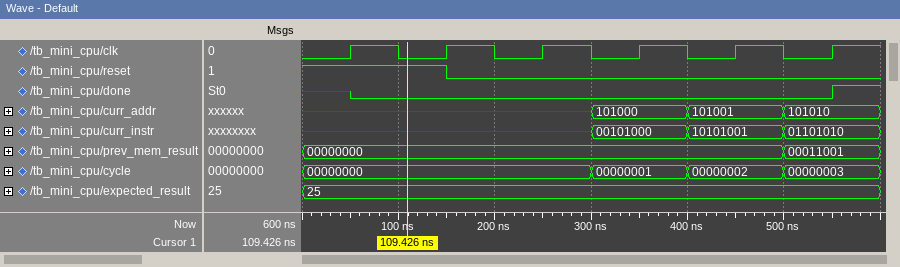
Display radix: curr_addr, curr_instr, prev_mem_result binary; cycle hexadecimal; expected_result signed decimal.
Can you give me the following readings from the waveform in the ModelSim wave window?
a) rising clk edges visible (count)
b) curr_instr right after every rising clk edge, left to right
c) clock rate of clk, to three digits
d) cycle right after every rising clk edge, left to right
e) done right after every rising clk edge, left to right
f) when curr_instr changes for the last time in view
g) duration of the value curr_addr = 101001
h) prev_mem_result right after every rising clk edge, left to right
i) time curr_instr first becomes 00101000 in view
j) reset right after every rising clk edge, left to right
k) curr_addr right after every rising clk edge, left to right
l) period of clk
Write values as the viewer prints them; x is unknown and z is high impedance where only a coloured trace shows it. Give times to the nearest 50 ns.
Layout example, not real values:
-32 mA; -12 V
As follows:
6; x, x, x, 00101000, 10101001, 01101010; 10.0 MHz; 00000000, 00000000, 00000000, 00000001, 00000002, 00000003; 0 0 0 0 0 1; 500 ns; 100 ns; 00000000, 00000000, 00000000, 00000000, 00000000, 00011001; 300 ns; 1 0 0 0 0 0; x, x, x, 101000, 101001, 101010; 100 ns
